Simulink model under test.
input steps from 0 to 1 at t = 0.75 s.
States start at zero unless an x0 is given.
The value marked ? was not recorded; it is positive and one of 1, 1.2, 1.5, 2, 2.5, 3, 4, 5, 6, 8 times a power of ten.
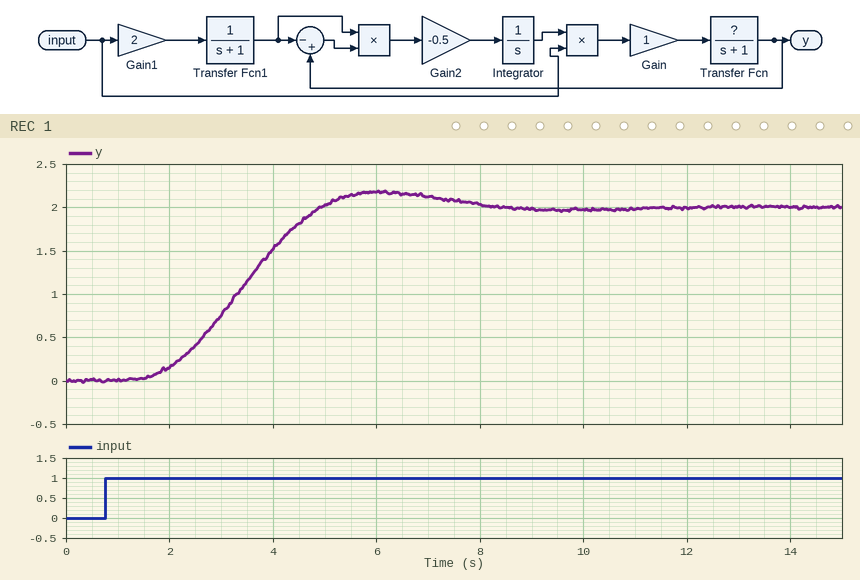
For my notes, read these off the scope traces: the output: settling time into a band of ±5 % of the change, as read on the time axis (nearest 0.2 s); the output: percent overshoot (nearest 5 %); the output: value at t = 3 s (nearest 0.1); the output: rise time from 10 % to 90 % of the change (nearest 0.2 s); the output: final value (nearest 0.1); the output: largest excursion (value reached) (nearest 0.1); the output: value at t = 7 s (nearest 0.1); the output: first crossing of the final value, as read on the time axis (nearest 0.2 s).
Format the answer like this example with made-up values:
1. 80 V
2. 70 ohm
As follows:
1. 7.2 s
2. 10 %
3. 0.8
4. 2.4 s
5. 2.0
6. 2.2
7. 2.1
8. 5.0 s
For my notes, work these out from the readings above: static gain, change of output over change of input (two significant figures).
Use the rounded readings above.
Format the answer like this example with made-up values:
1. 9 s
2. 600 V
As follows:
1. 2.0
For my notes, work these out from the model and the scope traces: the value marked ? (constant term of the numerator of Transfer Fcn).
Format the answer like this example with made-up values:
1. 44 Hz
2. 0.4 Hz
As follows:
1. 1
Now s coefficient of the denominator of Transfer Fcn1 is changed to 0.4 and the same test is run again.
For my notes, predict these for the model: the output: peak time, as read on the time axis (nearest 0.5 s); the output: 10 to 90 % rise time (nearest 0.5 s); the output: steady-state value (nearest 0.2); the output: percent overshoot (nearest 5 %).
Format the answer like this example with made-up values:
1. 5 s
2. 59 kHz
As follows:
1. 5.0 s
2. 2.0 s
3. 2.0
4. 15 %
